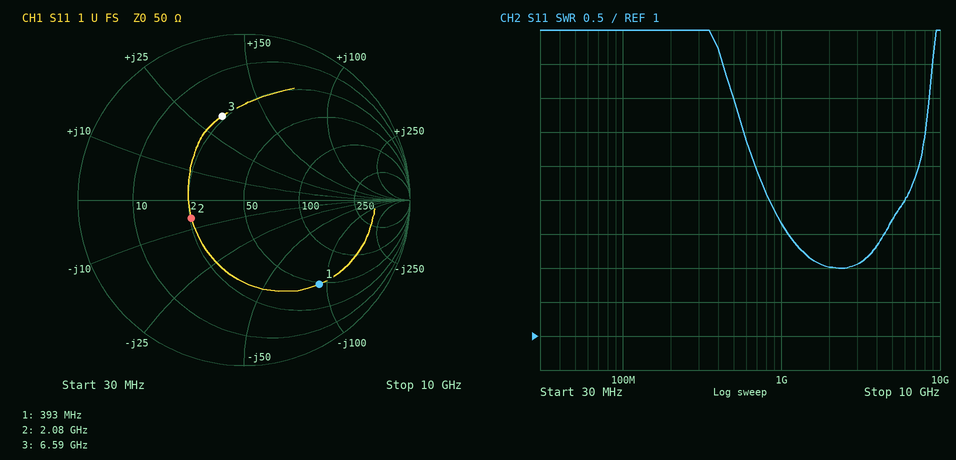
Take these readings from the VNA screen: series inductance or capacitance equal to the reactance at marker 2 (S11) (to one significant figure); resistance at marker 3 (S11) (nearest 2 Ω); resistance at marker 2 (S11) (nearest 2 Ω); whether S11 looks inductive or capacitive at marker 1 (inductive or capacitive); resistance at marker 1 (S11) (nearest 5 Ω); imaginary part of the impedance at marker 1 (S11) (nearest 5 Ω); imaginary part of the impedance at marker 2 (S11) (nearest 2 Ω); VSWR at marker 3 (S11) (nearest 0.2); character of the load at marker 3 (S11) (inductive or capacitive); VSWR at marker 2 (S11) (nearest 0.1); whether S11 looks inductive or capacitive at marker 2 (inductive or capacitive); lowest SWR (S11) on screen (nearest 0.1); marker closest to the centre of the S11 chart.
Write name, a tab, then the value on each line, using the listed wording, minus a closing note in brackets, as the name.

series inductance or capacitance equal to the reactance at marker 2 (S11)	10 pF
resistance at marker 3 (S11)	24 Ω
resistance at marker 2 (S11)	26 Ω
whether S11 looks inductive or capacitive at marker 1	capacitive
resistance at marker 1 (S11)	50 Ω
imaginary part of the impedance at marker 1 (S11)	-90 Ω
imaginary part of the impedance at marker 2 (S11)	-6 Ω
VSWR at marker 3 (S11)	3.2
character of the load at marker 3 (S11)	inductive
VSWR at marker 2 (S11)	2.0
whether S11 looks inductive or capacitive at marker 2	capacitive
lowest SWR (S11) on screen	2.0
marker closest to the centre of the S11 chart	marker 2
